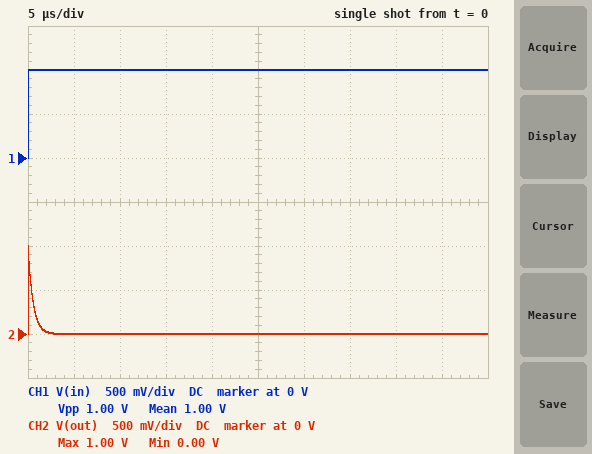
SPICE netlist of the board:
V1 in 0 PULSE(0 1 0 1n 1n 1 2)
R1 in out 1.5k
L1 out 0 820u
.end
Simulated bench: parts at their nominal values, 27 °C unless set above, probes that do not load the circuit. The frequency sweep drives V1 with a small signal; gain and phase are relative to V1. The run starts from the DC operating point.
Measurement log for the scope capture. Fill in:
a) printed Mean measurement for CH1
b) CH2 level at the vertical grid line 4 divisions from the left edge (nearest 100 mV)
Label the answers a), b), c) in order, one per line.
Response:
a) 1.00 V
b) 0 V
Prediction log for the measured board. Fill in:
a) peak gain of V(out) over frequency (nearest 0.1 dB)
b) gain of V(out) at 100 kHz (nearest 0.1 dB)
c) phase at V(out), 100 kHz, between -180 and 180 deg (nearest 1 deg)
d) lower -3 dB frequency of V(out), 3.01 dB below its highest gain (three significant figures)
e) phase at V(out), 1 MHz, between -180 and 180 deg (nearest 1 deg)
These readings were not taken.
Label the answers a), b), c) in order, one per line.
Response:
a) 0 dB
b) -9.8 dB
c) 71 deg
d) 291 kHz
e) 16 deg
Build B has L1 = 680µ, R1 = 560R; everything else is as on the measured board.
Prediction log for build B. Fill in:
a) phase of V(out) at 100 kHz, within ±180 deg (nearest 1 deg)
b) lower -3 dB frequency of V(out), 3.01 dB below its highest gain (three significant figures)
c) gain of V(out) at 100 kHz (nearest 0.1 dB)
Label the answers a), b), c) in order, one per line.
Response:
a) 53 deg
b) 131 kHz
c) -4.3 dB
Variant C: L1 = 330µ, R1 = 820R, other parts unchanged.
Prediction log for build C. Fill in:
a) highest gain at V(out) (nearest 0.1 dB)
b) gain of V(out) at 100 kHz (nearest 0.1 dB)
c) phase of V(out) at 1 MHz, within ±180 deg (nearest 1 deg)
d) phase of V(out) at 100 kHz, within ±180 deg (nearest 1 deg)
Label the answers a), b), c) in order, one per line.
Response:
a) 0 dB
b) -12.2 dB
c) 22 deg
d) 76 deg
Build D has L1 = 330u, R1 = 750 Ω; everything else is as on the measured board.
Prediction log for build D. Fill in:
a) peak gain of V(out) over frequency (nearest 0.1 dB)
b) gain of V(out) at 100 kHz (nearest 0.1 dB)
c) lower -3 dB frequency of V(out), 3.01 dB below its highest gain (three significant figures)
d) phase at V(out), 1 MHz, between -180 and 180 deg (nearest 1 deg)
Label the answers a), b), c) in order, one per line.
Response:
a) 0 dB
b) -11.5 dB
c) 362 kHz
d) 20 deg
